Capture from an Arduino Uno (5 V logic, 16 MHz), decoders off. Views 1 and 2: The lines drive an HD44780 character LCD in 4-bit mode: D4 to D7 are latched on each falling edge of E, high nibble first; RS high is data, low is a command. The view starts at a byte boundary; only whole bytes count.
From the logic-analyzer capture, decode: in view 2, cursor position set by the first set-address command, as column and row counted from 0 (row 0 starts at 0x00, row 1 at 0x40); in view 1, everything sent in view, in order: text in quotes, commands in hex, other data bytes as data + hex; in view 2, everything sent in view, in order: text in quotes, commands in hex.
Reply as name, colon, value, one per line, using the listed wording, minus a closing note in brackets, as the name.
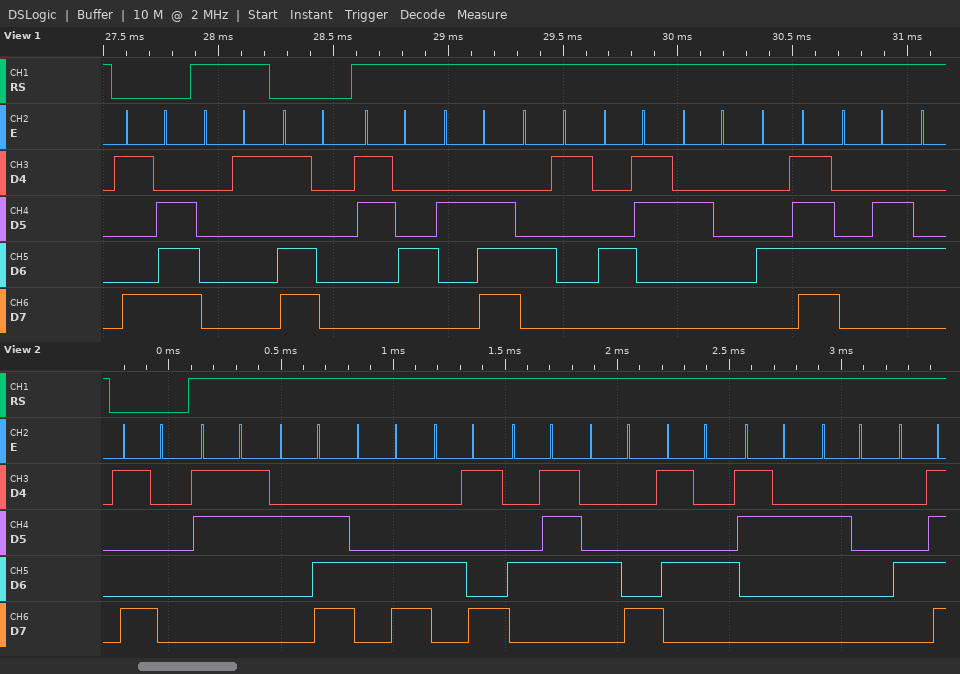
in view 2, cursor position set by the first set-address command, as column and row counted from 0: column 16, row 0
in view 1, everything sent in view, in order: text in quotes, commands in hex, other data bytes as data + hex: 0x9E data 01 0xD0 "4.AC OF"
in view 2, everything sent in view, in order: text in quotes, commands in hex: 0x90 "3.LIGHT2 O"
